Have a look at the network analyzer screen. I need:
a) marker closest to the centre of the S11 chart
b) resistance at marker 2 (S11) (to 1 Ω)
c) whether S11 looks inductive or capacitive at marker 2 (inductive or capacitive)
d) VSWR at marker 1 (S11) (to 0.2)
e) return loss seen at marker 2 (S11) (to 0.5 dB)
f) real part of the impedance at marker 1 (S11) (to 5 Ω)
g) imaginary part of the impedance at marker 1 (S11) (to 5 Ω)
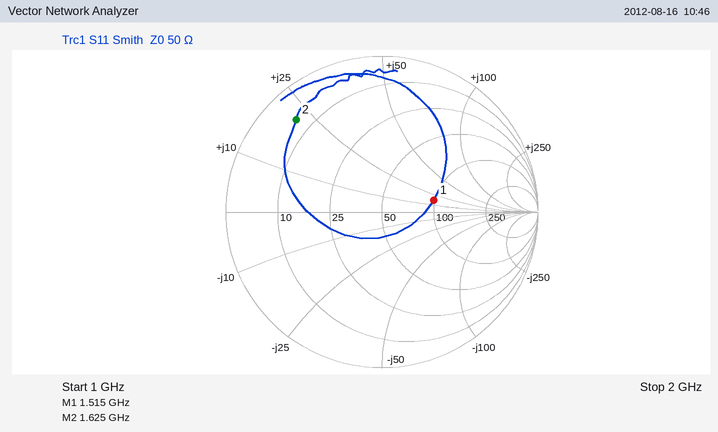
marker 1
6 Ω
inductive
2.0
2.0 dB
100 Ω
+15 Ω
